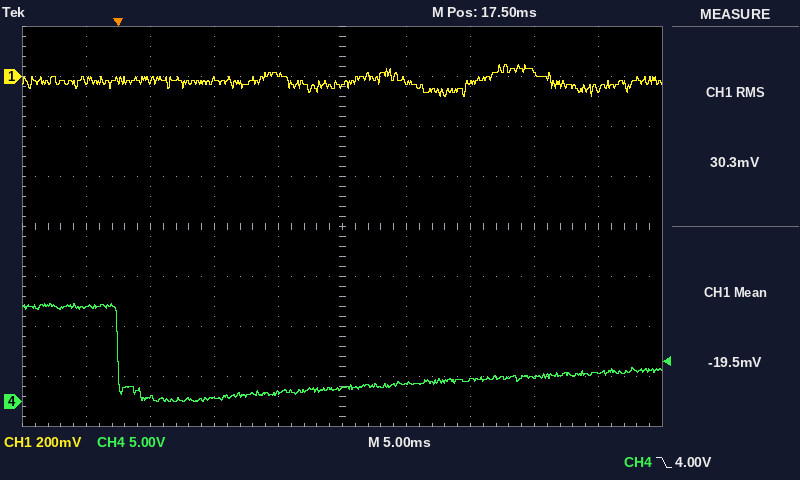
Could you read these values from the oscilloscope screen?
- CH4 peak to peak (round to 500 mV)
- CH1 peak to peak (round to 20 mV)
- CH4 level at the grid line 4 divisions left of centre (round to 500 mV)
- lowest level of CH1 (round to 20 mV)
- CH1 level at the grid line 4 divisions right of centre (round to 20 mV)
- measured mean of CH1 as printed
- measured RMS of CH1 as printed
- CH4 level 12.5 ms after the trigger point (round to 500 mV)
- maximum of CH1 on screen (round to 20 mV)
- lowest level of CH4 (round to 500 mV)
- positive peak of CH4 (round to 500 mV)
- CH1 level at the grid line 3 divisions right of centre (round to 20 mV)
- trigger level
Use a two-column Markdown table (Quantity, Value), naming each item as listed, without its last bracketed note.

| Quantity | Value |
|---|---|
| CH4 peak to peak | 10.0 V |
| CH1 peak to peak | 120 mV |
| CH4 level at the grid line 4 divisions left of centre | 9.5 V |
| lowest level of CH1 | -80 mV |
| CH1 level at the grid line 4 divisions right of centre | -40 mV |
| measured mean of CH1 as printed | -19.5 mV |
| measured RMS of CH1 as printed | 30.3 mV |
| CH4 level 12.5 ms after the trigger point | 1.0 V |
| maximum of CH1 on screen | 40 mV |
| lowest level of CH4 | 0.0 V |
| positive peak of CH4 | 10.0 V |
| CH1 level at the grid line 3 divisions right of centre | 20 mV |
| trigger level | 4.00 V |
